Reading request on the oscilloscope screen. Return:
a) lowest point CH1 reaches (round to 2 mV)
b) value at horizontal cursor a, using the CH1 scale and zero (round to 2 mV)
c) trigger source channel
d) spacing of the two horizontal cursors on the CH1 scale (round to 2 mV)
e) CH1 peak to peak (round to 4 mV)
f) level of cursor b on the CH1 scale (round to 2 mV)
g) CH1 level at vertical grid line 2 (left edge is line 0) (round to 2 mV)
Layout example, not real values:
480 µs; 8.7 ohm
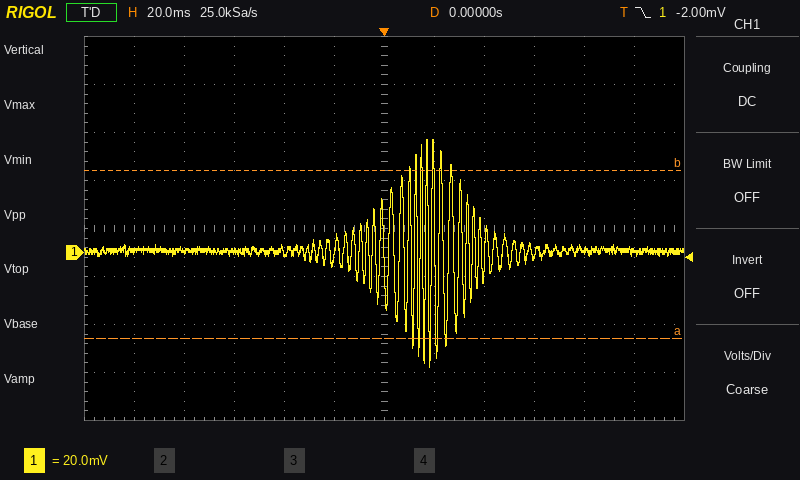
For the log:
-48 mV; -36 mV; CH1; 70 mV; 96 mV; 34 mV; 0 mV
